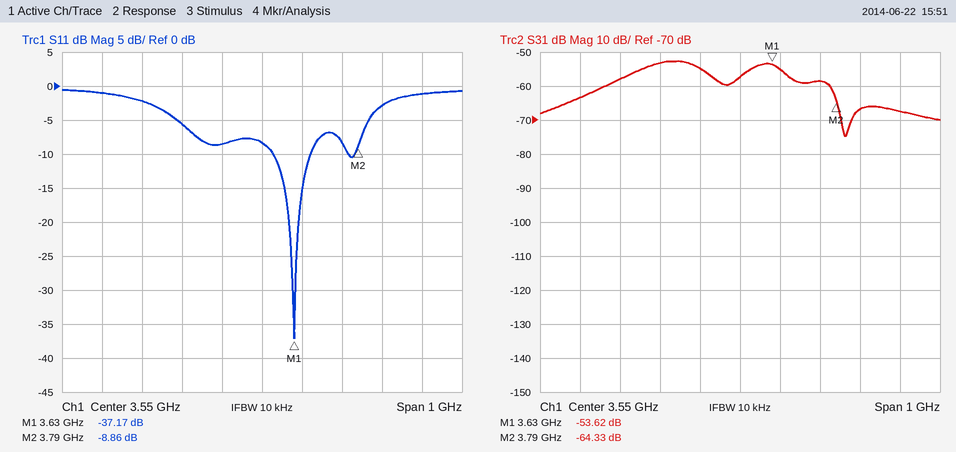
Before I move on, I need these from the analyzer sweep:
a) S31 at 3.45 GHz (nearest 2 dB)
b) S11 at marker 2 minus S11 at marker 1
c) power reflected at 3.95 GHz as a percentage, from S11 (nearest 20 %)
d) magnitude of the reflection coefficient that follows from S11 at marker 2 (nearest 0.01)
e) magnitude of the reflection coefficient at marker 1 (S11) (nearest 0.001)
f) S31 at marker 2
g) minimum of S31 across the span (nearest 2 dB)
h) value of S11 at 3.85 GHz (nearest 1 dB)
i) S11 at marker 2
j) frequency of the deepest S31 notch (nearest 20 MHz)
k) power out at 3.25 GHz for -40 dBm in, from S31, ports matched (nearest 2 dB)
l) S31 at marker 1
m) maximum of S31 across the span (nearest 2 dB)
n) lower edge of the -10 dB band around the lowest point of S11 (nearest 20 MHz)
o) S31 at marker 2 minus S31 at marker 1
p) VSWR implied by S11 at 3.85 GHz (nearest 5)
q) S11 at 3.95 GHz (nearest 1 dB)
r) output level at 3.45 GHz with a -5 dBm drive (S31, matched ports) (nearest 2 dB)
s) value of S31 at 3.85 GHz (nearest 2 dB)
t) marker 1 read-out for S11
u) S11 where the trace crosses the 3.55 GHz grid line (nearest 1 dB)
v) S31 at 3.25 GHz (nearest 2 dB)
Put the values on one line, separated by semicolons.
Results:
-54 dB; 28.31 dB; 80 %; 0.36; 0.014; -64.33 dB; -74 dB; -3 dB; -8.86 dB; 3.82 GHz; -98 dBm; -53.62 dB; -52 dB; 3.58 GHz; -10.71 dB; 5; -1 dB; -60 dBm; -66 dB; -37.17 dB; -8 dB; -58 dB
